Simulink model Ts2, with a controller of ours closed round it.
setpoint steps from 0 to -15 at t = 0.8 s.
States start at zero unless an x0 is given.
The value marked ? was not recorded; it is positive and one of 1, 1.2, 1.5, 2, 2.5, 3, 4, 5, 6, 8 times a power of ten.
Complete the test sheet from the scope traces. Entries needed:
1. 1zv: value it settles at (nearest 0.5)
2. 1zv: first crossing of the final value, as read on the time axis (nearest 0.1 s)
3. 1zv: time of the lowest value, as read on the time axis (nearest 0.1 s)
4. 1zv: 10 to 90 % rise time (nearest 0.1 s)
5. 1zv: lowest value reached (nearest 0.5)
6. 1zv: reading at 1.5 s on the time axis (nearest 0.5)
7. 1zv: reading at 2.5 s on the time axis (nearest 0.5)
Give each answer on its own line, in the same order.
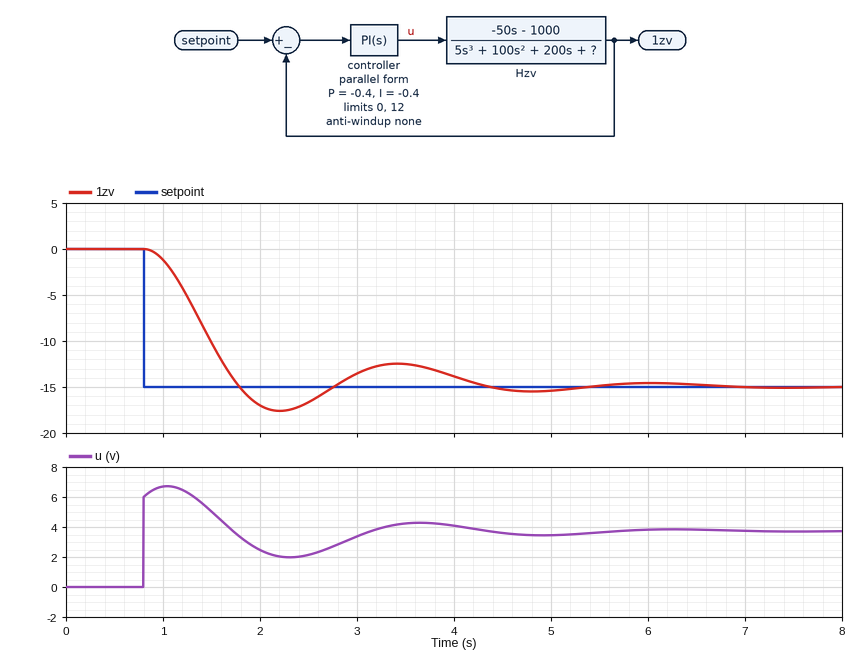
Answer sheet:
-15.0
1.8 s
2.2 s
0.7 s
-17.5
-10.0
-16.5
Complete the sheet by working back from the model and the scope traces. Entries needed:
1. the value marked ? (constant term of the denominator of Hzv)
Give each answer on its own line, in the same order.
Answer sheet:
250
